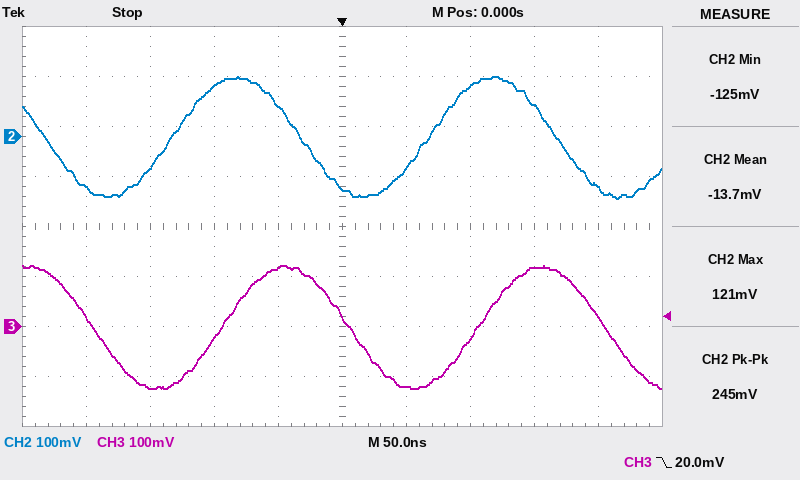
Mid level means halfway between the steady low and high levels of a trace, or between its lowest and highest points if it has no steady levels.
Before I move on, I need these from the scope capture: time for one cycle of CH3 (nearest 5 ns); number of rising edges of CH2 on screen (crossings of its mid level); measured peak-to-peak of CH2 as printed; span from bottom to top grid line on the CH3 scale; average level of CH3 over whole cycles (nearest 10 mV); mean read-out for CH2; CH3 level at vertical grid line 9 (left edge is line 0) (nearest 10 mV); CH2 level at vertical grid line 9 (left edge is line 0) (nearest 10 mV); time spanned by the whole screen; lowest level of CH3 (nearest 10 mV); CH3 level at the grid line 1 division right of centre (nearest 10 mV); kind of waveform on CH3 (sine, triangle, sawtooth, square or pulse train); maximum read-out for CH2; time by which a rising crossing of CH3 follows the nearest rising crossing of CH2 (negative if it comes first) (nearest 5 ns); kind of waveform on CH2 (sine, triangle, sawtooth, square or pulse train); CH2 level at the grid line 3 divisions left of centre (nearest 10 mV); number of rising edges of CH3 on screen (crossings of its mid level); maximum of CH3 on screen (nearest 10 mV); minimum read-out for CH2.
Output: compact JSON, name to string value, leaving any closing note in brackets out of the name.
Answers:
{"time for one cycle of CH3": "200 ns", "number of rising edges of CH2 on screen": "2", "measured peak-to-peak of CH2 as printed": "245 mV", "span from bottom to top grid line on the CH3 scale": "800 mV", "average level of CH3 over whole cycles": "0 mV", "mean read-out for CH2": "-13.7 mV", "CH3 level at vertical grid line 9 (left edge is line 0)": "20 mV", "CH2 level at vertical grid line 9 (left edge is line 0)": "-100 mV", "time spanned by the whole screen": "500 ns", "lowest level of CH3": "-120 mV", "CH3 level at the grid line 1 division right of centre": "-120 mV", "kind of waveform on CH3": "sine", "maximum read-out for CH2": "121 mV", "time by which a rising crossing of CH3 follows the nearest rising crossing of CH2 (negative if it comes first)": "+40 ns", "kind of waveform on CH2": "sine", "CH2 level at the grid line 3 divisions left of centre": "-60 mV", "number of rising edges of CH3 on screen": "2", "maximum of CH3 on screen": "120 mV", "minimum read-out for CH2": "-125 mV"}
